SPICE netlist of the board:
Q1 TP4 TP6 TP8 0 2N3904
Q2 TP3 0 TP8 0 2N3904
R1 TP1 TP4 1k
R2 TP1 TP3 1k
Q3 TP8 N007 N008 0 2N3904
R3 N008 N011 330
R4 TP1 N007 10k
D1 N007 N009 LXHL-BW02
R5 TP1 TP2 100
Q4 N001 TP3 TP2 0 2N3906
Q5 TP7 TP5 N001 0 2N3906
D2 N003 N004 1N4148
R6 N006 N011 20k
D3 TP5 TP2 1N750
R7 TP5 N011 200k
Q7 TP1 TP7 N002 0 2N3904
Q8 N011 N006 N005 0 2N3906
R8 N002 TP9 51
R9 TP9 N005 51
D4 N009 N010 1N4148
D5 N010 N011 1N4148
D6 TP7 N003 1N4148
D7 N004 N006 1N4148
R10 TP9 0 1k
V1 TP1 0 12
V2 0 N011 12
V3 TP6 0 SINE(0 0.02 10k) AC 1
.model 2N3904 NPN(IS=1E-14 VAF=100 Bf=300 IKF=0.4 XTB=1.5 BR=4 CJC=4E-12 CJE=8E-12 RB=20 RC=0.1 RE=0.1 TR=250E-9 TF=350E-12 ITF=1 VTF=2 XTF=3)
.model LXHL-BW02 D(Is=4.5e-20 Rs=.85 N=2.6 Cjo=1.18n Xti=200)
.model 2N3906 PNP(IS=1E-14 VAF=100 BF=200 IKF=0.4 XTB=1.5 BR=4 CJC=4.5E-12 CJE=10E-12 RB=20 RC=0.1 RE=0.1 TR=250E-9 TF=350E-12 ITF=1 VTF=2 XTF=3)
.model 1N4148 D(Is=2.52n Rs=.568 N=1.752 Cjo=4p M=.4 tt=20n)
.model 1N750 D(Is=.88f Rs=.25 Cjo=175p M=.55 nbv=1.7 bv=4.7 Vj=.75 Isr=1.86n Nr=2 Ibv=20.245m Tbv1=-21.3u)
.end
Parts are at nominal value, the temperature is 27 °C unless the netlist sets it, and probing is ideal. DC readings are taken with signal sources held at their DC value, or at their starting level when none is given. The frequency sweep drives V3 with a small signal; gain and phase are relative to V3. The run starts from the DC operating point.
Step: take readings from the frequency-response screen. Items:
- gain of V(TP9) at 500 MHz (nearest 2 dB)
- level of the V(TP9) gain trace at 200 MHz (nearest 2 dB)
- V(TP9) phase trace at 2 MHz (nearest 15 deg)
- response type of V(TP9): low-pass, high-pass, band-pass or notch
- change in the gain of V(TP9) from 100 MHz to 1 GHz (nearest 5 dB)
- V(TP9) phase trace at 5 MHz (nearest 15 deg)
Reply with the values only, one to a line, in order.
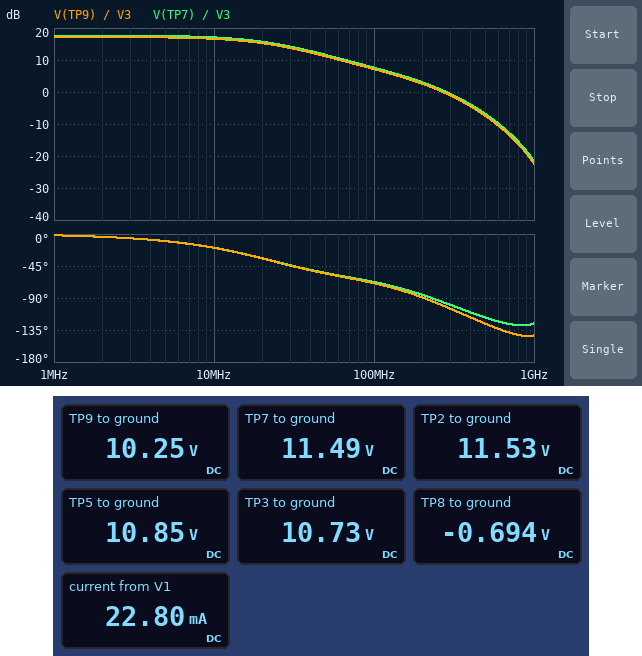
-8 dB
2 dB
0 deg
low-pass
-30 dB
-15 deg
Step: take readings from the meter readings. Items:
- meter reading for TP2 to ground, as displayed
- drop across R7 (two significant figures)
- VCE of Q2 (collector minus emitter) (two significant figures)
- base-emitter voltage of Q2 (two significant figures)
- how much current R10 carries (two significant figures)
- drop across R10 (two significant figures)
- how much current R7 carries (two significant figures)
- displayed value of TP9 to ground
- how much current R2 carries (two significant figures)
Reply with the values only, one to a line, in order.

11.53 V
23 V
11 V
690 mV
10 mA
10 V
110 µA
10.25 V
1.3 mA
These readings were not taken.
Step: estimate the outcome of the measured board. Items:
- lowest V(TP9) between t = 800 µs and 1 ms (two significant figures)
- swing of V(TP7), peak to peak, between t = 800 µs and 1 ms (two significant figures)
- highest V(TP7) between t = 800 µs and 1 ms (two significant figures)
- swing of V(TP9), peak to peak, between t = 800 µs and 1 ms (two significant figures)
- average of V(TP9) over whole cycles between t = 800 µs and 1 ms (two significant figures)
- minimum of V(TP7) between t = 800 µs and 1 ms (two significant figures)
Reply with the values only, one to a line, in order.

10 V
290 mV
12 V
270 mV
10 V
11 V
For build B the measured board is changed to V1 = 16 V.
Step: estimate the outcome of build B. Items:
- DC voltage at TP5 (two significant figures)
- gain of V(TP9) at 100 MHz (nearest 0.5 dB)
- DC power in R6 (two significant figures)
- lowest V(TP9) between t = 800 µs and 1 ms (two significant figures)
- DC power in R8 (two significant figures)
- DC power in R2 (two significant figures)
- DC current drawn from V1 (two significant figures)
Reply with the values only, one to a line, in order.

15 V
7.5 dB
33 mW
14 V
10 mW
1.7 mW
27 mA
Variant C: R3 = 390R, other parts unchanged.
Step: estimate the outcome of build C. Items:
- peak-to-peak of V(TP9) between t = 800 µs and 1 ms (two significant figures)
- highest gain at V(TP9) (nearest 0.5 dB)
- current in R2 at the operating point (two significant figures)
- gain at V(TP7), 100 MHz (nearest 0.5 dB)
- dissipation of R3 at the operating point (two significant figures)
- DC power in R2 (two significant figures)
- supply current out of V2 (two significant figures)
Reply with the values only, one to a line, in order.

230 mV
16.0 dB
1.2 mA
7.0 dB
25 mW
1.4 mW
11 mA
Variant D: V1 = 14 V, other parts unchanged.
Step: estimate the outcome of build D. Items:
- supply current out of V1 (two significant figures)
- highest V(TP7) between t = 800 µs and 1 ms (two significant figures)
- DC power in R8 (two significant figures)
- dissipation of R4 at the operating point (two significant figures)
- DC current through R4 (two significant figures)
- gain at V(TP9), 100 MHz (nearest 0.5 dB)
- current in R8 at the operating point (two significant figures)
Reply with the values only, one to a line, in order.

25 mA
14 V
7.5 mW
49 mW
2.2 mA
7.5 dB
12 mA
